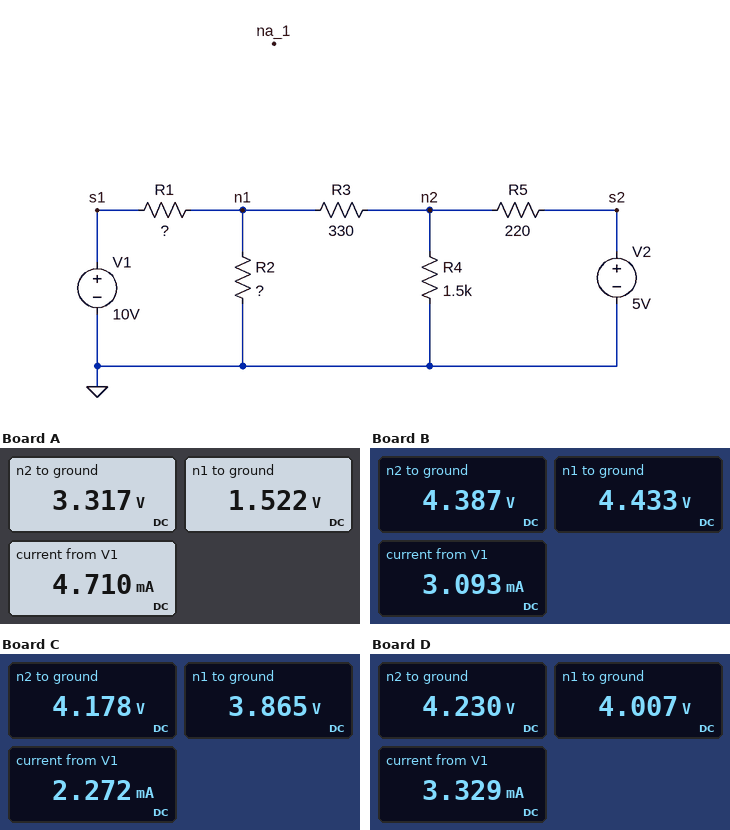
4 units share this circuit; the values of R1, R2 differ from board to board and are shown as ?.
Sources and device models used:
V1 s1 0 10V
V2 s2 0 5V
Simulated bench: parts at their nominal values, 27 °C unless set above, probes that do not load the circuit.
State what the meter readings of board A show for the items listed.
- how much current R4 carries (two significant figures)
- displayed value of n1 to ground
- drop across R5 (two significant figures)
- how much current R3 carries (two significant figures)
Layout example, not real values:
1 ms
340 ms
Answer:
2.2 mA
1.522 V
1.7 V
5.4 mA
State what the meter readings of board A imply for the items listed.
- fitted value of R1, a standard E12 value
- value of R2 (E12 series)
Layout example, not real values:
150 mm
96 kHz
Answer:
1.8 kΩ
150 Ω
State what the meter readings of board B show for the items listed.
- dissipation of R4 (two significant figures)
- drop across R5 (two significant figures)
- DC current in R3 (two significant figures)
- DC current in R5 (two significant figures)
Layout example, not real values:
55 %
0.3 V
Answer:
13 mW
610 mV
140 µA
2.8 mA
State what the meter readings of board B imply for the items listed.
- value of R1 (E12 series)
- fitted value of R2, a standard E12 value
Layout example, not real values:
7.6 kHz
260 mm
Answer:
1.8 kΩ
1.5 kΩ
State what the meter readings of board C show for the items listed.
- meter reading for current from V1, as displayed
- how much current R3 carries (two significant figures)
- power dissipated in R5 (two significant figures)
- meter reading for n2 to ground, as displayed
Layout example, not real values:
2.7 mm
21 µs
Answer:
2.272 mA
950 µA
3.1 mW
4.178 V
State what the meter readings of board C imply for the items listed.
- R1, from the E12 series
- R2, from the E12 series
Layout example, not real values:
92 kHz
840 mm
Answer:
2.7 kΩ
1.2 kΩ
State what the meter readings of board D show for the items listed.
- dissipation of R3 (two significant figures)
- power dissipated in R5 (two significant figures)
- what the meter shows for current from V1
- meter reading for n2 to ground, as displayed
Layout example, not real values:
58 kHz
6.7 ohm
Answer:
150 µW
2.7 mW
3.329 mA
4.230 V
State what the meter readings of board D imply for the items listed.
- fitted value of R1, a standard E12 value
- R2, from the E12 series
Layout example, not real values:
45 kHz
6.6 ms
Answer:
1.8 kΩ
1 kΩ
